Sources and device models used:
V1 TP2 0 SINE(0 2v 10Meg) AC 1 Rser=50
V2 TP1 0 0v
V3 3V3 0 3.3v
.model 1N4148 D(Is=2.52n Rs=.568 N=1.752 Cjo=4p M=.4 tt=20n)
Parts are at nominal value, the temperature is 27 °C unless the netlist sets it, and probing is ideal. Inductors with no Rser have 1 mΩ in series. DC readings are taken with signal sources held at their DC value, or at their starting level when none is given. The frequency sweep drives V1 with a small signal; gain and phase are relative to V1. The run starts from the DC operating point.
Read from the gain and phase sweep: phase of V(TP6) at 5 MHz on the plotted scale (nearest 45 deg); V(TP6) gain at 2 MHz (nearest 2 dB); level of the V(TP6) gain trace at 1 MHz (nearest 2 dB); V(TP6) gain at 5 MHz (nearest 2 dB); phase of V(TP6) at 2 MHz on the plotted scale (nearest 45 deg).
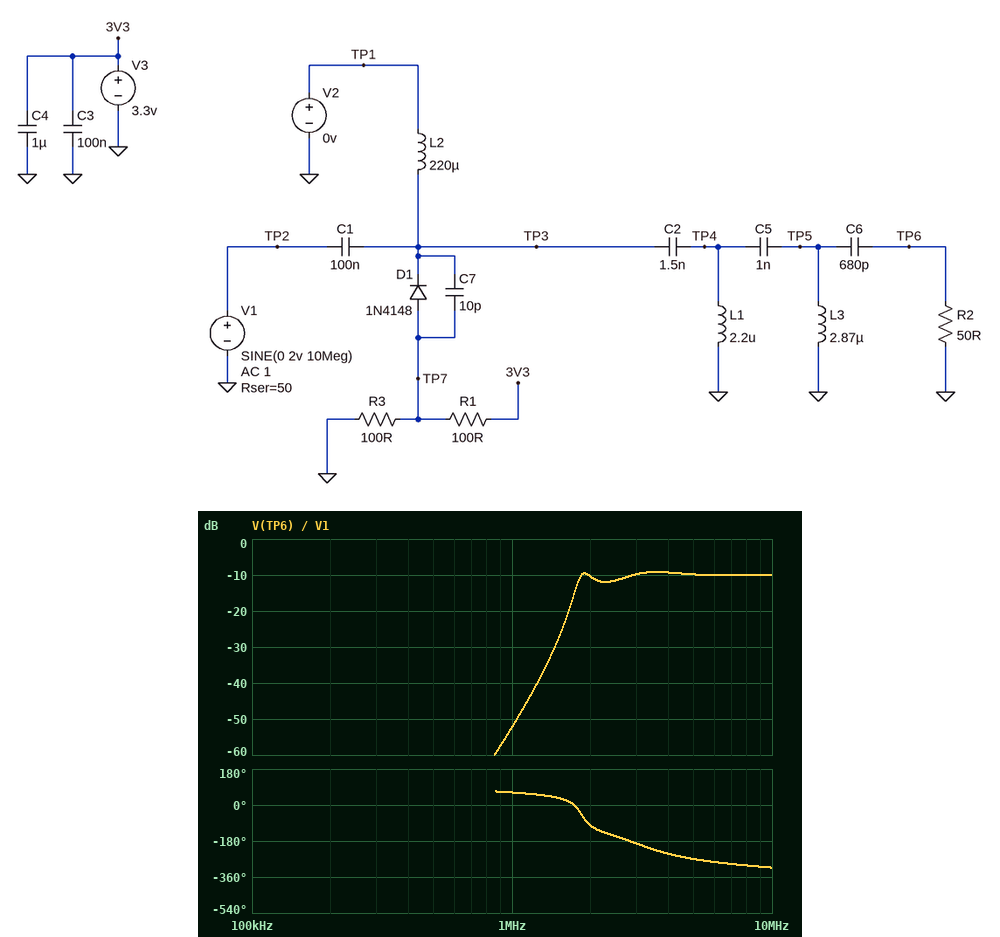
-270 deg
-10 dB
-52 dB
-10 dB
-90 deg
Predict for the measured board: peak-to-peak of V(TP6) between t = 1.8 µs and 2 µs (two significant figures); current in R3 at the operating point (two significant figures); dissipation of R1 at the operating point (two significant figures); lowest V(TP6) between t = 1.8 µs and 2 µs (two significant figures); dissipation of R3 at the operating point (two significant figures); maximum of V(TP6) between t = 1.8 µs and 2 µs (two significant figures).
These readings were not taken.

1.3 V
7.3 mA
66 mW
-640 mV
5.3 mW
630 mV
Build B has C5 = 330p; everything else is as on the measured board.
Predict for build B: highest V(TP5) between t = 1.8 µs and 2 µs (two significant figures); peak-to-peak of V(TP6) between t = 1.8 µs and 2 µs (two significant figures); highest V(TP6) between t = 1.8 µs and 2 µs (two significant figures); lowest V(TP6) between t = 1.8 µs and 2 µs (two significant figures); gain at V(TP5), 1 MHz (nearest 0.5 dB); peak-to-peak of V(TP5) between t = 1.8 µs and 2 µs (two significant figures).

600 mV
1.1 V
550 mV
-550 mV
-50.0 dB
1.2 V
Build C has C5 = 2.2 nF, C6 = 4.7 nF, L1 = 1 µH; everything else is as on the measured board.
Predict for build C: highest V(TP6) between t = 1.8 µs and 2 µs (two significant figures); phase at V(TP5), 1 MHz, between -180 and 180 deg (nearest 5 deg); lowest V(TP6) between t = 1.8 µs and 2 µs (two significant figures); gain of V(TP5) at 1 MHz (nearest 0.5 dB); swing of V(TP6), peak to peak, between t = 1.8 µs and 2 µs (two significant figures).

690 mV
-35 deg
-690 mV
-37.0 dB
1.4 V
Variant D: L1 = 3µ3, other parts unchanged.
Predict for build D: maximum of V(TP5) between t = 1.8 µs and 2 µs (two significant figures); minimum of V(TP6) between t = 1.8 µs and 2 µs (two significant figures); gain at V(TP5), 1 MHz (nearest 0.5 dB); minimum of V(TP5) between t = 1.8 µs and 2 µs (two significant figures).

690 mV
-620 mV
-34.0 dB
-690 mV
